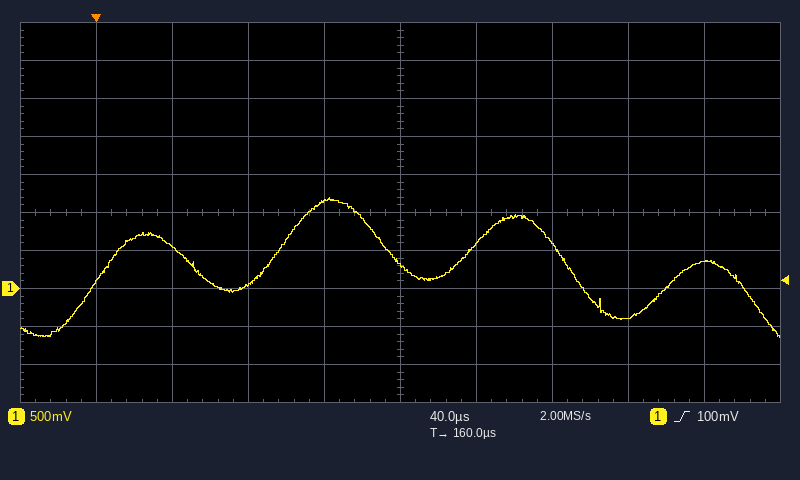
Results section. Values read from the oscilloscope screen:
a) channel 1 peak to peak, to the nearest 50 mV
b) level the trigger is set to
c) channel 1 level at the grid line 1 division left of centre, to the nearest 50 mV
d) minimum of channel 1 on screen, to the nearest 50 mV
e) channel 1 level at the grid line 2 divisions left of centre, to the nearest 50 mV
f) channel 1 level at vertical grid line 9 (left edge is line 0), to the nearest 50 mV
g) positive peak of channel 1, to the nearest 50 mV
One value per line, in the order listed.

1.85 V
100 mV
1.15 V
-650 mV
50 mV
350 mV
1.20 V
